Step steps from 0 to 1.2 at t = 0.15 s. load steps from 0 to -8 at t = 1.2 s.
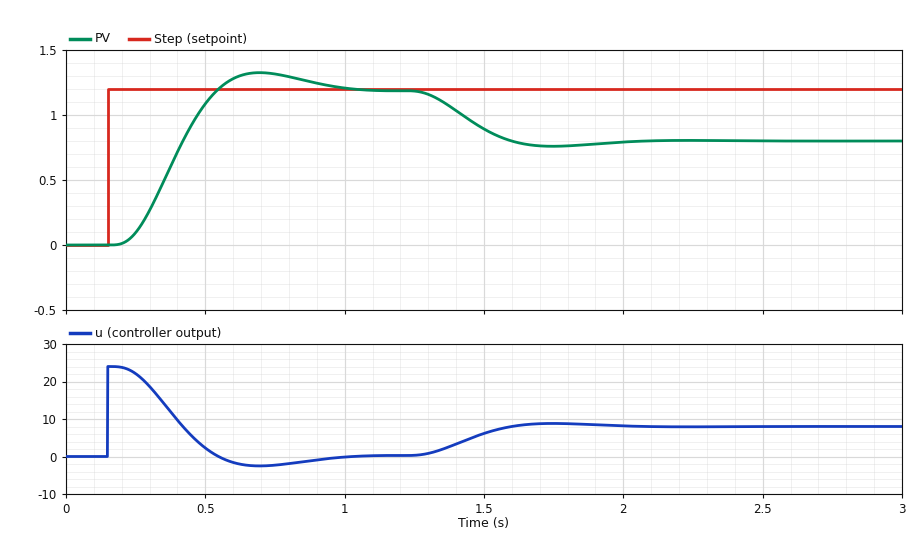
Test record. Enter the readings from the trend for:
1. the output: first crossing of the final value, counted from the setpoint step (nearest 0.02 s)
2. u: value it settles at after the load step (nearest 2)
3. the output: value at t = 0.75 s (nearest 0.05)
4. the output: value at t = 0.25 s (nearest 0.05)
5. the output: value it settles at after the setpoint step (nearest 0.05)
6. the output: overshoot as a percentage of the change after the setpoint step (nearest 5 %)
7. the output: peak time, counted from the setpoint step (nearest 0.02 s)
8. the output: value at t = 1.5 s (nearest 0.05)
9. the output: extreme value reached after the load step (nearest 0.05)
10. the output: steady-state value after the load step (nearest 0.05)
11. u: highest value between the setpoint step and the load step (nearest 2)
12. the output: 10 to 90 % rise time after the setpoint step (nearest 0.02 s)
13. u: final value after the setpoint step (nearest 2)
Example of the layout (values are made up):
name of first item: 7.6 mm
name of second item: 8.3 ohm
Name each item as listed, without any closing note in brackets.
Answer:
the output: first crossing of the final value, counted from the setpoint step: 0.40 s
u: value it settles at after the load step: 8
the output: value at t = 0.75 s: 1.30
the output: value at t = 0.25 s: 0.10
the output: value it settles at after the setpoint step: 1.20
the output: overshoot as a percentage of the change after the setpoint step: 10 %
the output: peak time, counted from the setpoint step: 0.54 s
the output: value at t = 1.5 s: 0.90
the output: extreme value reached after the load step: 0.75
the output: steady-state value after the load step: 0.80
u: highest value between the setpoint step and the load step: 24
the output: 10 to 90 % rise time after the setpoint step: 0.24 s
u: final value after the setpoint step: 0
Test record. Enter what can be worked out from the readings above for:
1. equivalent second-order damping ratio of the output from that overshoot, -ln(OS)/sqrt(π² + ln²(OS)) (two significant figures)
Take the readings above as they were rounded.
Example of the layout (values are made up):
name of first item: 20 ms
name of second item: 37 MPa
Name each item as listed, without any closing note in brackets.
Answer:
equivalent second-order damping ratio of the output from that overshoot, -ln(OS)/sqrt(π² + ln²(OS)): 0.59
